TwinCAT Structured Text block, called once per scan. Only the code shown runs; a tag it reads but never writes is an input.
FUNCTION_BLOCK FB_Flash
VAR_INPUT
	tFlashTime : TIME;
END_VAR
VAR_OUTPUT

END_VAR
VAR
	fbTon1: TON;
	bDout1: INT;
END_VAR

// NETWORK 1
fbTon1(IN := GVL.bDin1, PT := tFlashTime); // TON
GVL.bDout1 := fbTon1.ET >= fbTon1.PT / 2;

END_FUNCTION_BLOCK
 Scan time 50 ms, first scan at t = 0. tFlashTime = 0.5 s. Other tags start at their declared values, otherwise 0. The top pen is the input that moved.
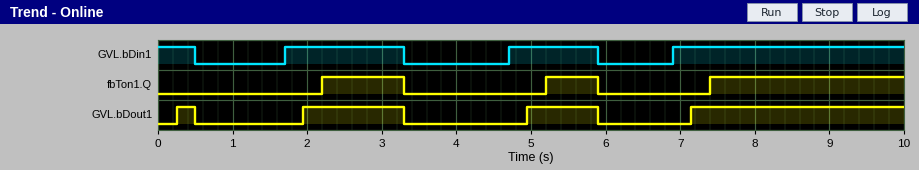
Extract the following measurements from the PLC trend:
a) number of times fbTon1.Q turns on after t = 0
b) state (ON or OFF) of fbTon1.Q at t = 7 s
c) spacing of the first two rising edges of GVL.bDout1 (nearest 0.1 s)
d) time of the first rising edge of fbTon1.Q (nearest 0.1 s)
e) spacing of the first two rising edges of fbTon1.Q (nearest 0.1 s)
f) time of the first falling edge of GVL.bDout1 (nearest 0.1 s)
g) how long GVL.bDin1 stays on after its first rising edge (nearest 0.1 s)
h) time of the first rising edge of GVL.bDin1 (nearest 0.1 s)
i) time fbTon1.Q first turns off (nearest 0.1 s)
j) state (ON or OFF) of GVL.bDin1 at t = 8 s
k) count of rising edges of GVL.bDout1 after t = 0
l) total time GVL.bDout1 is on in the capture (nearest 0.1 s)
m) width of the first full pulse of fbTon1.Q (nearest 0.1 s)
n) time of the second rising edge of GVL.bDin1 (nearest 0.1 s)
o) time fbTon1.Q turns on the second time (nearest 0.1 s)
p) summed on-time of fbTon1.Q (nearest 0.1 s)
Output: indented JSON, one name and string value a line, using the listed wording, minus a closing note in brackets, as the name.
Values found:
{
  "number of times fbTon1.Q turns on after t = 0": "3",
  "state (ON or OFF) of fbTon1.Q at t = 7 s": "OFF",
  "spacing of the first two rising edges of GVL.bDout1": "1.7 s",
  "time of the first rising edge of fbTon1.Q": "2.2 s",
  "spacing of the first two rising edges of fbTon1.Q": "3.0 s",
  "time of the first falling edge of GVL.bDout1": "0.5 s",
  "how long GVL.bDin1 stays on after its first rising edge": "1.6 s",
  "time of the first rising edge of GVL.bDin1": "1.7 s",
  "time fbTon1.Q first turns off": "3.3 s",
  "state (ON or OFF) of GVL.bDin1 at t = 8 s": "ON",
  "count of rising edges of GVL.bDout1 after t = 0": "4",
  "total time GVL.bDout1 is on in the capture": "5.4 s",
  "width of the first full pulse of fbTon1.Q": "1.1 s",
  "time of the second rising edge of GVL.bDin1": "4.7 s",
  "time fbTon1.Q turns on the second time": "5.2 s",
  "summed on-time of fbTon1.Q": "4.4 s"
}
